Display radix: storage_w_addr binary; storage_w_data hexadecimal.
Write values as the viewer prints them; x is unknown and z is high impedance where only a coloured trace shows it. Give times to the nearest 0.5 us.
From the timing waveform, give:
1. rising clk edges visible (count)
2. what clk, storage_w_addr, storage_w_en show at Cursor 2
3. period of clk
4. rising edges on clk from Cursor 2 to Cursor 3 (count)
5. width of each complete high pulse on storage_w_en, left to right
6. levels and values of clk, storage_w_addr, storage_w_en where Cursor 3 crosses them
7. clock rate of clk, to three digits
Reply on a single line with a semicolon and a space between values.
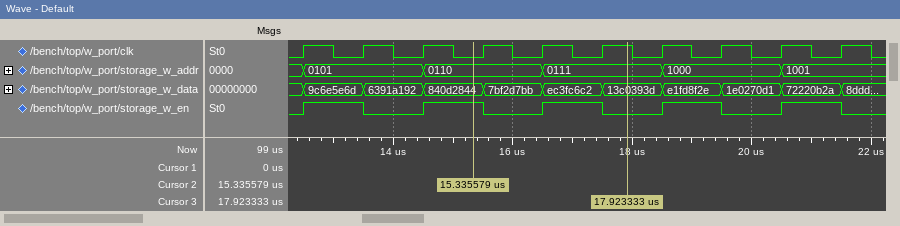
10; clk=0, storage_w_addr=0110, storage_w_en=1; 1 us; 3; 1 us, 1 us, 1 us, 1 us, 1 us; clk=1, storage_w_addr=0111, storage_w_en=0; 1.00 MHz
